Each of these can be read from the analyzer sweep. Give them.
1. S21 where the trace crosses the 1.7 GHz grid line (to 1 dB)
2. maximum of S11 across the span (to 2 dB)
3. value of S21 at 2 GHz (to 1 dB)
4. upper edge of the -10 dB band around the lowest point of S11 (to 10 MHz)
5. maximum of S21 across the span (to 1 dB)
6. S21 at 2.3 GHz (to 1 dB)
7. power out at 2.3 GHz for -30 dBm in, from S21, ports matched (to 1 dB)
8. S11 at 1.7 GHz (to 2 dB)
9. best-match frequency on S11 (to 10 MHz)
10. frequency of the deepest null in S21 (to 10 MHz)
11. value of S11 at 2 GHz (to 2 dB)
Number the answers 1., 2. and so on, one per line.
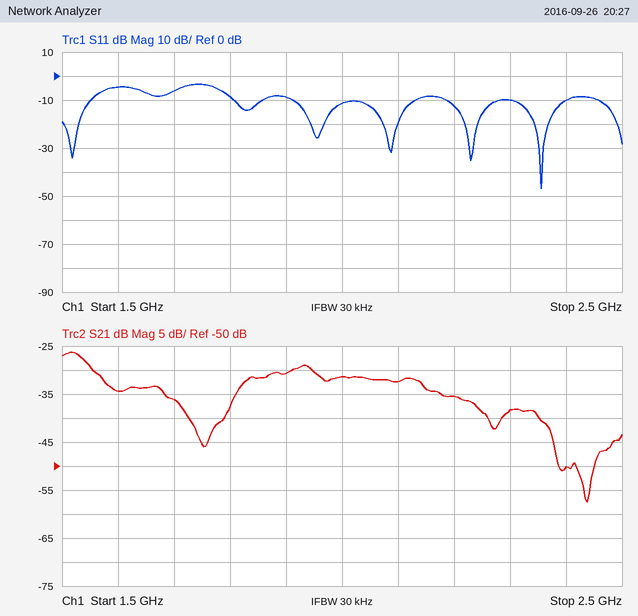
1. -36 dB
2. -4 dB
3. -31 dB
4. 2.40 GHz
5. -26 dB
6. -38 dB
7. -68 dBm
8. -6 dB
9. 2.36 GHz
10. 2.44 GHz
11. -12 dB
